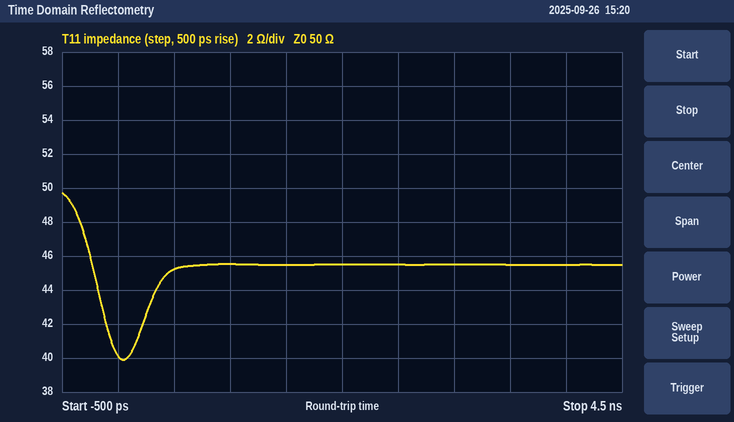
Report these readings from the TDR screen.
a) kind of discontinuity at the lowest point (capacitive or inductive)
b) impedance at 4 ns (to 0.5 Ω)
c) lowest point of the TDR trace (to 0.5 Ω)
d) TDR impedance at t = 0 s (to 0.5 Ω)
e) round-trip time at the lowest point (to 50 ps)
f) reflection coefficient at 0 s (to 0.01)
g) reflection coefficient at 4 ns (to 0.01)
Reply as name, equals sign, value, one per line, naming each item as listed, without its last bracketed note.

kind of discontinuity at the lowest point = capacitive
impedance at 4 ns = 45.5 Ω
lowest point of the TDR trace = 40.0 Ω
TDR impedance at t = 0 s = 40.0 Ω
round-trip time at the lowest point = 50 ps
reflection coefficient at 0 s = -0.11
reflection coefficient at 4 ns = -0.05
